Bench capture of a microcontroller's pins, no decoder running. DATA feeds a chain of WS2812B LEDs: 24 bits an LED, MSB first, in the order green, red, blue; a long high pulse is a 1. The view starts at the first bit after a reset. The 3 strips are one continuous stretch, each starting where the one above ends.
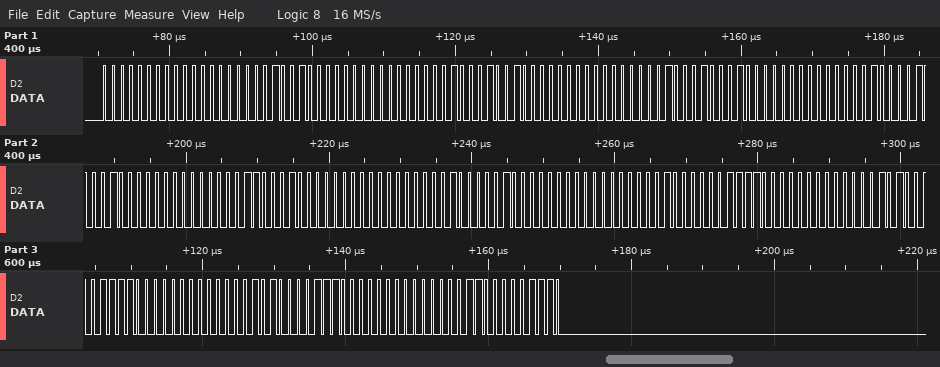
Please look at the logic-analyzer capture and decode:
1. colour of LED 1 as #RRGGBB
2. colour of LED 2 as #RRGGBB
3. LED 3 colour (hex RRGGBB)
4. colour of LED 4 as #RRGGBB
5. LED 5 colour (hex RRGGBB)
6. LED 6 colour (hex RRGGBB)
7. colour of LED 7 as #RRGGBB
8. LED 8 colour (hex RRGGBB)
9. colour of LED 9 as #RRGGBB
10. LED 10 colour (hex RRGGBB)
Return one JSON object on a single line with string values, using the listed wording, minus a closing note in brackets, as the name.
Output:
{"colour of LED 1 as #RRGGBB": "#000012", "colour of LED 2 as #RRGGBB": "#010012", "LED 3 colour": "#010011", "colour of LED 4 as #RRGGBB": "#020011", "LED 5 colour": "#030010", "LED 6 colour": "#040010", "colour of LED 7 as #RRGGBB": "#04000F", "LED 8 colour": "#05000F", "colour of LED 9 as #RRGGBB": "#05000E", "LED 10 colour": "#06000E"}
